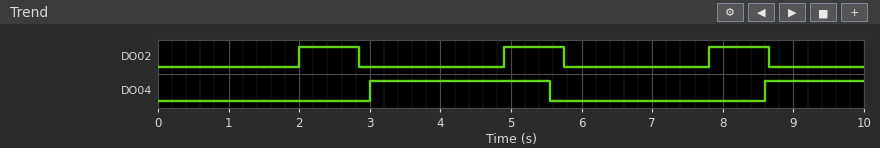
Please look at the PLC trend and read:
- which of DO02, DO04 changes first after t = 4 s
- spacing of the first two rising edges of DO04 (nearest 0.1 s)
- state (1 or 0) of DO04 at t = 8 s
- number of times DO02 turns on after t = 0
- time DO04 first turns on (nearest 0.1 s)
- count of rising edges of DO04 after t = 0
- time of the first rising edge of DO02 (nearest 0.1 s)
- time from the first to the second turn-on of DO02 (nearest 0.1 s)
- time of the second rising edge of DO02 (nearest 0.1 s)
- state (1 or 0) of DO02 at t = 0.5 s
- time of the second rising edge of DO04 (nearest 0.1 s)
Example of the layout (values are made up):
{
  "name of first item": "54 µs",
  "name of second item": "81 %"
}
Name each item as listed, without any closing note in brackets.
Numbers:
{
  "which of DO02, DO04 changes first after t = 4 s": "DO02",
  "spacing of the first two rising edges of DO04": "5.6 s",
  "state (1 or 0) of DO04 at t = 8 s": "0",
  "number of times DO02 turns on after t = 0": "3",
  "time DO04 first turns on": "3.0 s",
  "count of rising edges of DO04 after t = 0": "2",
  "time of the first rising edge of DO02": "2.0 s",
  "time from the first to the second turn-on of DO02": "2.9 s",
  "time of the second rising edge of DO02": "4.9 s",
  "state (1 or 0) of DO02 at t = 0.5 s": "0",
  "time of the second rising edge of DO04": "8.6 s"
}
